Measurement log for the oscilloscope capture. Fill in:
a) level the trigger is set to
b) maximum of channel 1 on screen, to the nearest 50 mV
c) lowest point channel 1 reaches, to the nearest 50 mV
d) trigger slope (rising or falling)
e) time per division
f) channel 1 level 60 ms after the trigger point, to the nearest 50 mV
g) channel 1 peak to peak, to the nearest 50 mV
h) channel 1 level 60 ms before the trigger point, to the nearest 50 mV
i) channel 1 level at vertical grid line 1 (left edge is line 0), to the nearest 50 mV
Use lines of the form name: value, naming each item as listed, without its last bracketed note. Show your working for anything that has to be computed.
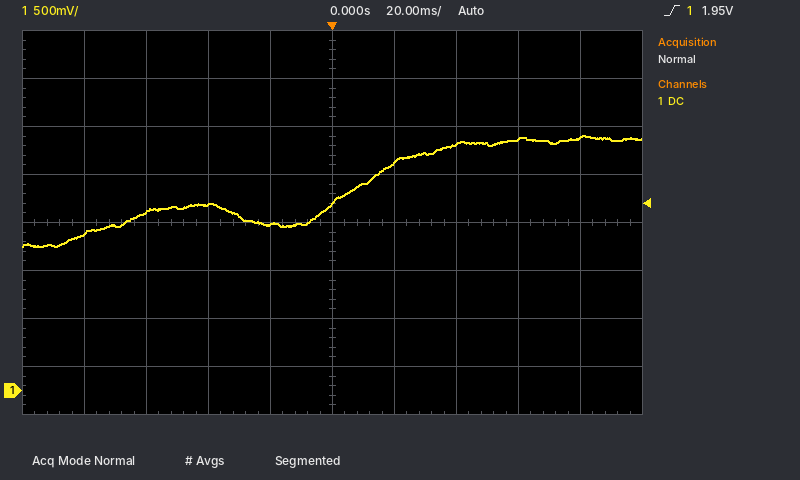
level the trigger is set to: 1.95 V
maximum of channel 1 on screen, to the nearest 50 mV: 2.65 V
lowest point channel 1 reaches, to the nearest 50 mV: 1.50 V
trigger slope: rising
time per division: 20 ms
channel 1 level 60 ms after the trigger point, to the nearest 50 mV: 2.60 V
channel 1 peak to peak, to the nearest 50 mV: 2.65 V − (1.50 V) = 1.15 V
channel 1 level 60 ms before the trigger point, to the nearest 50 mV: 1.85 V
channel 1 level at vertical grid line 1 (left edge is line 0), to the nearest 50 mV: 1.65 V
